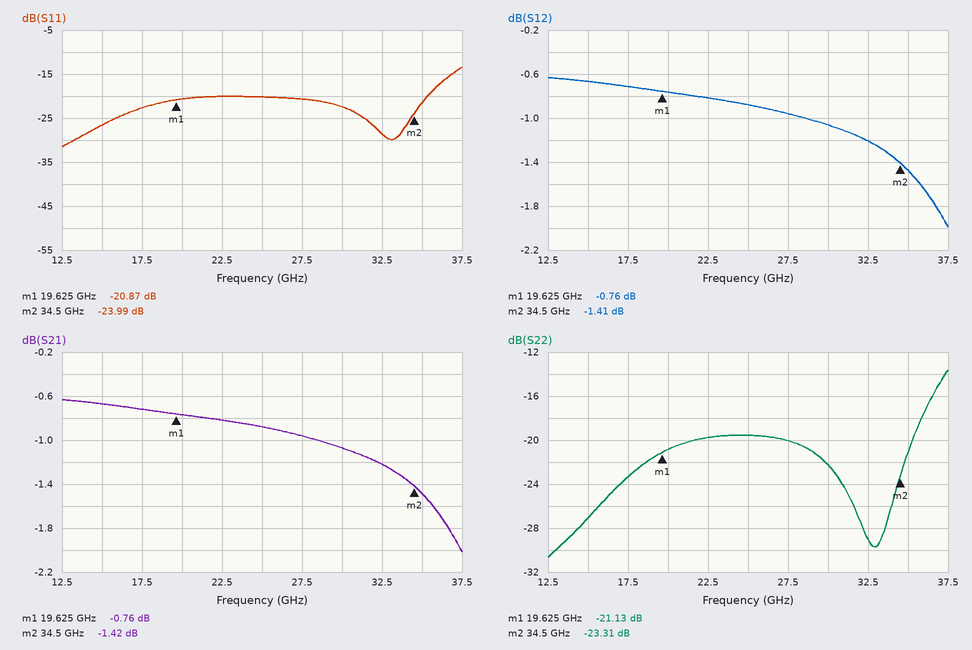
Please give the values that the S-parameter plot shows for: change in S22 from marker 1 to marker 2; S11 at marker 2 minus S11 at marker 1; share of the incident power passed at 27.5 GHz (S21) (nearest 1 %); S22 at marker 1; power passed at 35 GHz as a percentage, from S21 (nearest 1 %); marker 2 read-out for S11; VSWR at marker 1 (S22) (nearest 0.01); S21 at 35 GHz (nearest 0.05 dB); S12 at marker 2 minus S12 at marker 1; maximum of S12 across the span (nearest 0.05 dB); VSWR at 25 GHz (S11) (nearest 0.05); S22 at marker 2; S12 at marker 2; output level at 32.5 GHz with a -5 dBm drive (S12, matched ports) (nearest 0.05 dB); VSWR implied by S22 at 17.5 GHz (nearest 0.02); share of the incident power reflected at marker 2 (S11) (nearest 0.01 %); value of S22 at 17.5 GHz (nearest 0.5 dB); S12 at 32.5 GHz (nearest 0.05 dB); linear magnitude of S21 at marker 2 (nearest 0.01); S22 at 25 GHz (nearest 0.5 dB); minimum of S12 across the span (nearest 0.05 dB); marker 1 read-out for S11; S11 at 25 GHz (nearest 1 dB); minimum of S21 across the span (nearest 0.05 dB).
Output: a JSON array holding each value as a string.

["-2.18 dB", "-3.12 dB", "80 %", "-21.13 dB", "71 %", "-23.99 dB", "1.19", "-1.50 dB", "-0.65 dB", "-0.65 dB", "1.20", "-23.31 dB", "-1.41 dB", "-6.20 dBm", "1.14", "0.40 %", "-23.5 dB", "-1.20 dB", "0.85", "-19.5 dB", "-2.00 dB", "-20.87 dB", "-20 dB", "-2.00 dB"]
